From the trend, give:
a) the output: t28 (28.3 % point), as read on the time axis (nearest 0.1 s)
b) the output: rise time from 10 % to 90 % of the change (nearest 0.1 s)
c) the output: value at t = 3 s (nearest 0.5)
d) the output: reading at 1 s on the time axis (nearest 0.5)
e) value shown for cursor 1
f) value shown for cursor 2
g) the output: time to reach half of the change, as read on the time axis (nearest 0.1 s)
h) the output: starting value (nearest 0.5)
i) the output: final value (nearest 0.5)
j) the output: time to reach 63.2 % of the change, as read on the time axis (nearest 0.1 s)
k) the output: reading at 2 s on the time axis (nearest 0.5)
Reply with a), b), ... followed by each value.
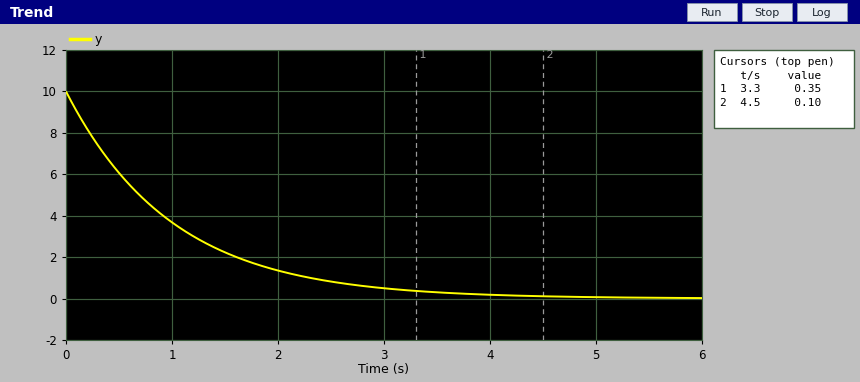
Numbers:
a) 0.3 s
b) 2.2 s
c) 0.5
d) 3.5
e) 0.35
f) 0.10
g) 0.7 s
h) 10.0
i) 0.0
j) 1.0 s
k) 1.5
